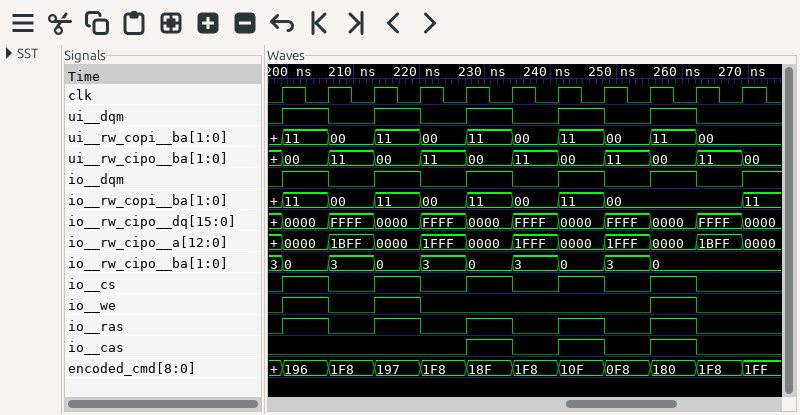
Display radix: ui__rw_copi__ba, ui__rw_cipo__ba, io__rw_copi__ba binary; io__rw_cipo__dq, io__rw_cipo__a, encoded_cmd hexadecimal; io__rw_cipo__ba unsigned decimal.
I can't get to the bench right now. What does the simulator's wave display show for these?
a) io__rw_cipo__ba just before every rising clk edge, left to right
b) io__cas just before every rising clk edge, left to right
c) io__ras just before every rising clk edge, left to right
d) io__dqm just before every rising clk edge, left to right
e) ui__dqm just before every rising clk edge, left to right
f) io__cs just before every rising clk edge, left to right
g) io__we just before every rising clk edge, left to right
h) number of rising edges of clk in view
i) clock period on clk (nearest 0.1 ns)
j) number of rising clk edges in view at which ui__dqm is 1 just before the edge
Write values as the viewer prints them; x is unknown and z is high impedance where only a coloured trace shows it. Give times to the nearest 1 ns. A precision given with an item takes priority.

3, 0, 3, 0, 3, 0, 3, 0, 3, 0, 0
0 0 0 0 0 1 0 1 0 1 0
0 1 0 1 0 1 0 1 0 1 0
0 1 0 1 0 1 0 1 0 1 0
0 1 0 1 0 1 0 1 0 1 0
0 1 0 1 0 1 0 1 0 1 0
0 1 0 1 0 0 0 0 0 1 0
11
7 ns
5
